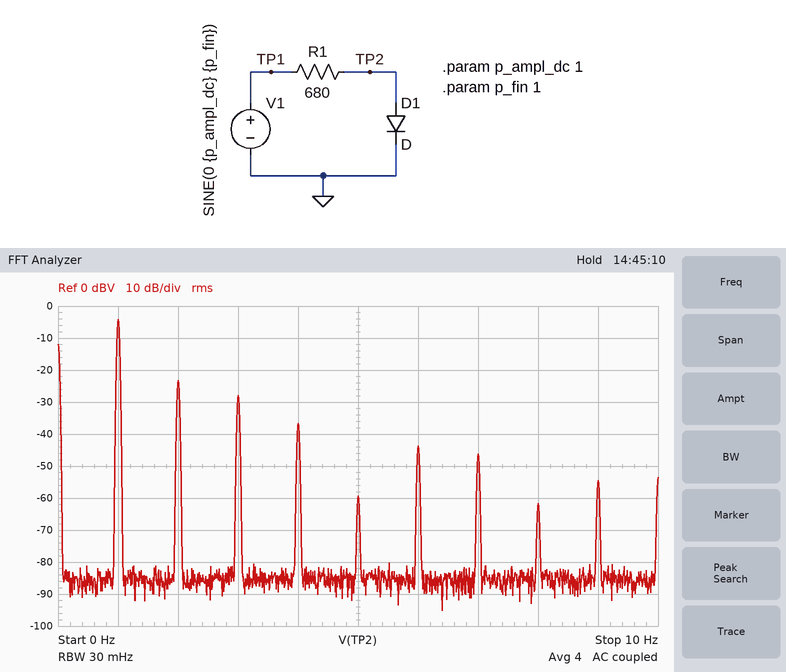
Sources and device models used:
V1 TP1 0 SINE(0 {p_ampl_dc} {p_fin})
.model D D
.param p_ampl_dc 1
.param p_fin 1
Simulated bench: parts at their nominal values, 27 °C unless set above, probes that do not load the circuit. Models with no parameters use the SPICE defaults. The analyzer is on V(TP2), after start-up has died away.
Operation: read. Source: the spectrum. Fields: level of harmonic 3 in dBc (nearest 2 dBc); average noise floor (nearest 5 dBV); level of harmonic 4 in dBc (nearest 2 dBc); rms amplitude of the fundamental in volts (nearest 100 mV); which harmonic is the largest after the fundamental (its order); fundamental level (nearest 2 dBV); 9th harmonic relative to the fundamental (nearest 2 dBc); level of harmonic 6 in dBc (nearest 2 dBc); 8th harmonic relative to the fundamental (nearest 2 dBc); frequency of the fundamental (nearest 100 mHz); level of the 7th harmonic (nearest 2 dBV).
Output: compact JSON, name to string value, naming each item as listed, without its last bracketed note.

{"level of harmonic 3 in dBc": "-24 dBc", "average noise floor": "-85 dBV", "level of harmonic 4 in dBc": "-32 dBc", "rms amplitude of the fundamental in volts": "600 mV", "which harmonic is the largest after the fundamental": "2", "fundamental level": "-4 dBV", "9th harmonic relative to the fundamental": "-50 dBc", "level of harmonic 6 in dBc": "-40 dBc", "8th harmonic relative to the fundamental": "-58 dBc", "frequency of the fundamental": "1.0 Hz", "level of the 7th harmonic": "-46 dBV"}
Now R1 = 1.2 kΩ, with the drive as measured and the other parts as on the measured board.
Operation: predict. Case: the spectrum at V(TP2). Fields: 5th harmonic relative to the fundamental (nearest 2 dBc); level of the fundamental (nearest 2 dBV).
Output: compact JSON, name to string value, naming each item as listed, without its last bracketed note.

{"5th harmonic relative to the fundamental": "-50 dBc", "level of the fundamental": "-4 dBV"}
